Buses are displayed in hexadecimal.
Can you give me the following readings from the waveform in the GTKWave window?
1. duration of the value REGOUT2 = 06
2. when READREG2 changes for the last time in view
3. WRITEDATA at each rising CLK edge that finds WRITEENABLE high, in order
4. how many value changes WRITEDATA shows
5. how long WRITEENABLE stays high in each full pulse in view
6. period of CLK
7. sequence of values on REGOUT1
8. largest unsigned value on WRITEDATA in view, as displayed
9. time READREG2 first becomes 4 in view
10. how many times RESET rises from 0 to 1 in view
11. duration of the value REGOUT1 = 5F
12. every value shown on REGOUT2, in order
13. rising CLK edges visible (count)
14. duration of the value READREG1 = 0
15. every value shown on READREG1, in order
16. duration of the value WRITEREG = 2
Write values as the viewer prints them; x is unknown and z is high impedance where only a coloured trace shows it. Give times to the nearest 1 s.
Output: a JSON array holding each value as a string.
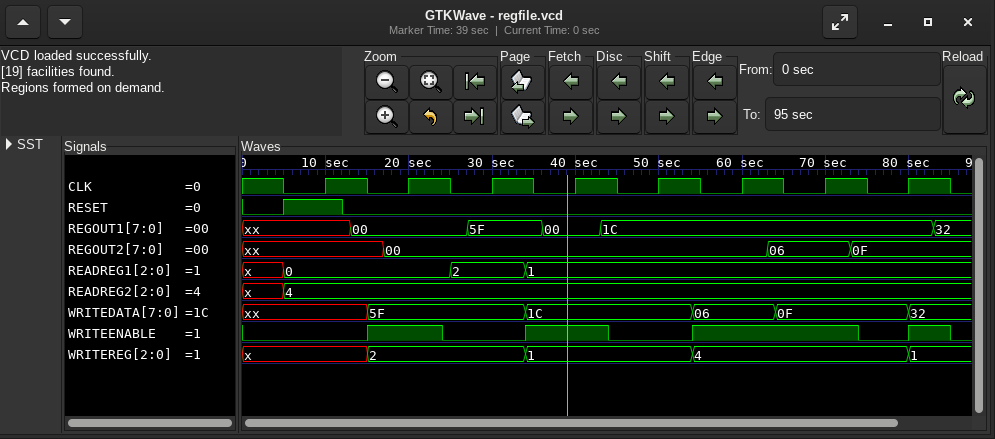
["10 s", "5 s", "5F, 1C, 06, 0F", "5", "9 s, 10 s, 20 s, 5 s", "10 s", "xx, 00, 5F, 00, 1C, 32", "5F", "5 s", "1", "9 s", "xx, 00, 06, 0F", "8", "20 s", "x, 0, 2, 1", "19 s"]
